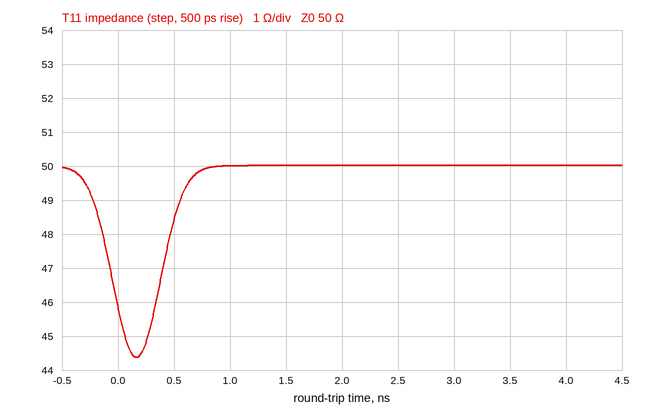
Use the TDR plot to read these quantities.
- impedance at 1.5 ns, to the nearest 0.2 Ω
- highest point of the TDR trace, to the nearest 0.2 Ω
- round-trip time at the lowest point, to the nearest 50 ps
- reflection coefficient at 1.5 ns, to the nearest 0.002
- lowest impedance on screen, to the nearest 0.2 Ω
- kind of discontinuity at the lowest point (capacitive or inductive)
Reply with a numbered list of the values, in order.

1. 50.0 Ω
2. 50.0 Ω
3. 150 ps
4. 0.000
5. 44.4 Ω
6. capacitive
